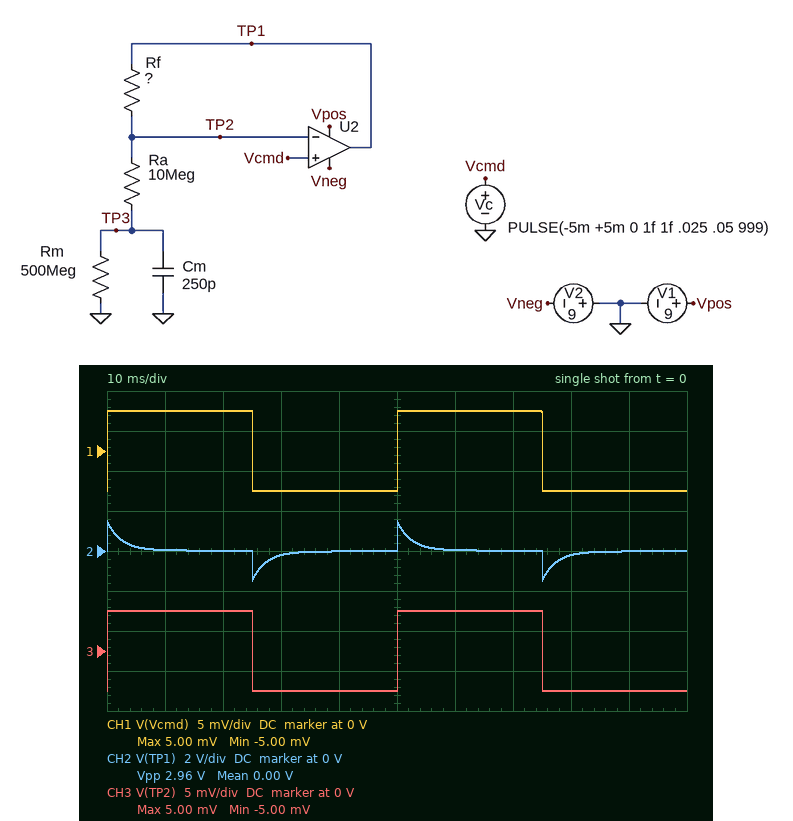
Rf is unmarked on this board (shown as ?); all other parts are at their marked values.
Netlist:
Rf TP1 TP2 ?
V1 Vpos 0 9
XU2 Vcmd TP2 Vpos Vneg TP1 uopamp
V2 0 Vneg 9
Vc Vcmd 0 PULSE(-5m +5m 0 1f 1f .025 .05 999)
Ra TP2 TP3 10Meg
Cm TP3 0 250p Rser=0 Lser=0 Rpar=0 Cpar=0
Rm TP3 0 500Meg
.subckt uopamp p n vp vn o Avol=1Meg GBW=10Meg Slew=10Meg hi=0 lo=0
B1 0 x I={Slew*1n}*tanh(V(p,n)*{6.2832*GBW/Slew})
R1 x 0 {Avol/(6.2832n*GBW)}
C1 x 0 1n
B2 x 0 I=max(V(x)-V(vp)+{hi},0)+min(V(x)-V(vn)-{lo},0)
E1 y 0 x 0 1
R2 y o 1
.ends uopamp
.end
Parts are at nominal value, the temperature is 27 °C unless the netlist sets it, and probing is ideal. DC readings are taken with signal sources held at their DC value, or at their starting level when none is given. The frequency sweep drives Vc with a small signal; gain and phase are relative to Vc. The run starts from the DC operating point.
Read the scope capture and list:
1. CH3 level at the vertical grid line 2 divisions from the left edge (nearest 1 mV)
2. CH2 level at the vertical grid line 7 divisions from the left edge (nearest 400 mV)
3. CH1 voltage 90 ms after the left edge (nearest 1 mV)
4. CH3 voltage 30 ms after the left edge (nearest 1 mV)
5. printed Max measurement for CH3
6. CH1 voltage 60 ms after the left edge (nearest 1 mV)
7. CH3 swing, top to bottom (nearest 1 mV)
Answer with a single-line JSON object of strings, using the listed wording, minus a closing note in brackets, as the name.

{"CH3 level at the vertical grid line 2 divisions from the left edge": "5 mV", "CH2 level at the vertical grid line 7 divisions from the left edge": "0 V", "CH1 voltage 90 ms after the left edge": "-5 mV", "CH3 voltage 30 ms after the left edge": "-5 mV", "printed Max measurement for CH3": "5.00 mV", "CH1 voltage 60 ms after the left edge": "5 mV", "CH3 swing, top to bottom": "10 mV"}
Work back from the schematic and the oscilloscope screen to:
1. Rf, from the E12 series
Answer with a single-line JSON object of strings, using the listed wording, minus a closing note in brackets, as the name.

{"Rf, from the E12 series": "1.5 GΩ"}
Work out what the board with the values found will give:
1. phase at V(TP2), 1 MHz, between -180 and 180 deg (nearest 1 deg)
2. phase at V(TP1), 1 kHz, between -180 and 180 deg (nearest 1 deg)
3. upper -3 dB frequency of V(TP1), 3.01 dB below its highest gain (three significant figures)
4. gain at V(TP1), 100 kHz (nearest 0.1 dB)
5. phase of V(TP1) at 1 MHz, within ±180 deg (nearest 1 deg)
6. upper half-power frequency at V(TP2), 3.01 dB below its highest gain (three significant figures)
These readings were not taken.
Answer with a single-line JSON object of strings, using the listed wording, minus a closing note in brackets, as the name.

{"phase at V(TP2), 1 MHz, between -180 and 180 deg": "-86 deg", "phase at V(TP1), 1 kHz, between -180 and 180 deg": "3 deg", "upper -3 dB frequency of V(TP1), 3.01 dB below its highest gain": "66.3 kHz", "gain at V(TP1), 100 kHz": "38.4 dB", "phase of V(TP1) at 1 MHz, within ±180 deg": "-86 deg", "upper half-power frequency at V(TP2), 3.01 dB below its highest gain": "66.2 kHz"}
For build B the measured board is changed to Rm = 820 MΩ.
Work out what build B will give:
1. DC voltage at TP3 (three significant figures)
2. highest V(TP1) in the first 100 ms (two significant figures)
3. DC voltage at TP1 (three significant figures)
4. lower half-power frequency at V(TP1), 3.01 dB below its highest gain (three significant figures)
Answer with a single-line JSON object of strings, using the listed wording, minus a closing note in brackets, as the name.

{"DC voltage at TP3": "-4.94 mV", "highest V(TP1) in the first 100 ms": "1.5 V", "DC voltage at TP1": "-14.0 mV", "lower half-power frequency at V(TP1), 3.01 dB below its highest gain": "64.3 Hz"}
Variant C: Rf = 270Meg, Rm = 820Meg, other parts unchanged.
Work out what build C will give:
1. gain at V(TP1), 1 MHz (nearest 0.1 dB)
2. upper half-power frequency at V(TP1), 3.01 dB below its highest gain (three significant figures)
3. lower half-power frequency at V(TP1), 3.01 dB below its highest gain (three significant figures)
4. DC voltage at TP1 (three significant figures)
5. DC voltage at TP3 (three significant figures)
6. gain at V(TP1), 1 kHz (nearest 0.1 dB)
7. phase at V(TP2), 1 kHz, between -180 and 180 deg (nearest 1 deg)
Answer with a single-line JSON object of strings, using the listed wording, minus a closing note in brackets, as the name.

{"gain at V(TP1), 1 MHz": "19.5 dB", "upper half-power frequency at V(TP1), 3.01 dB below its highest gain": "357 kHz", "lower half-power frequency at V(TP1), 3.01 dB below its highest gain": "64.3 Hz", "DC voltage at TP1": "-6.63 mV", "DC voltage at TP3": "-4.94 mV", "gain at V(TP1), 1 kHz": "28.9 dB", "phase at V(TP2), 1 kHz, between -180 and 180 deg": "0 deg"}
